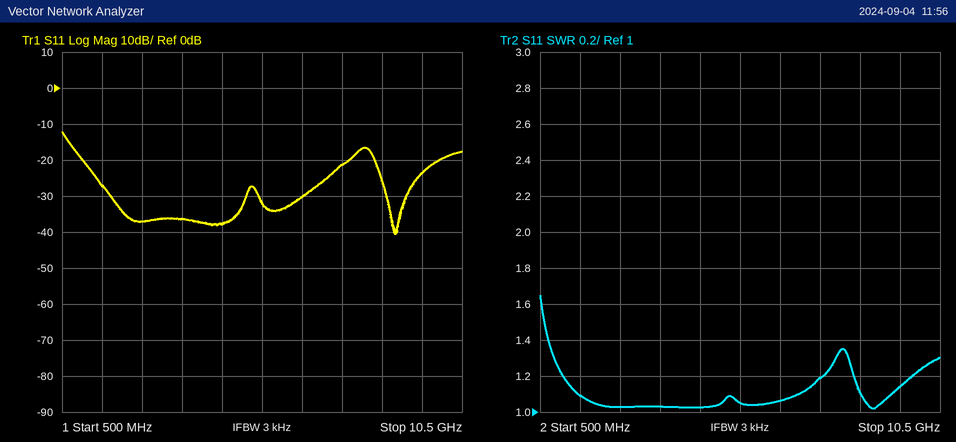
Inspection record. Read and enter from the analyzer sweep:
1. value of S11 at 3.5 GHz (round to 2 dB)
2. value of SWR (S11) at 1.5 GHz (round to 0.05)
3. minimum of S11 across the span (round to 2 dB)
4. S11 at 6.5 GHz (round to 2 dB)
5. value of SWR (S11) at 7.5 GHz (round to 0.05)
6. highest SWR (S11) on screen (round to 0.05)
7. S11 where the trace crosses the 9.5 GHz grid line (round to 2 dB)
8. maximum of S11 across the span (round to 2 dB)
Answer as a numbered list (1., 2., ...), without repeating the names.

1. -36 dB
2. 1.10
3. -40 dB
4. -30 dB
5. 1.20
6. 1.65
7. -24 dB
8. -12 dB
